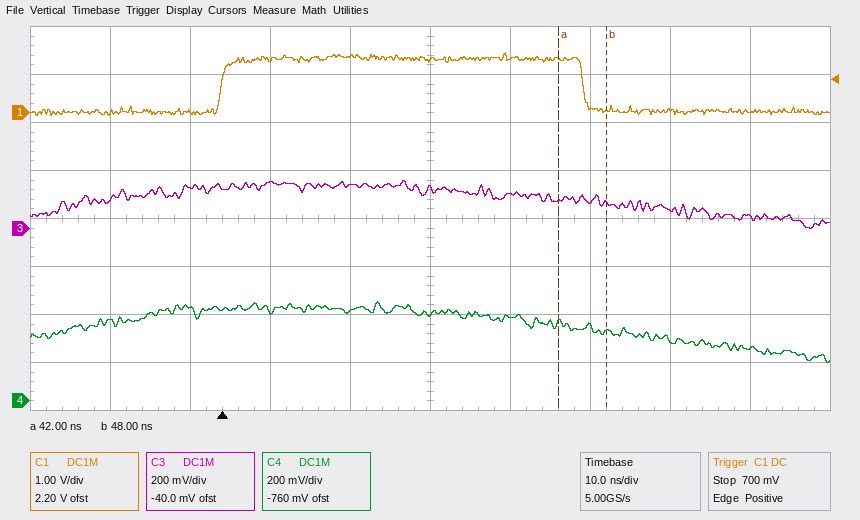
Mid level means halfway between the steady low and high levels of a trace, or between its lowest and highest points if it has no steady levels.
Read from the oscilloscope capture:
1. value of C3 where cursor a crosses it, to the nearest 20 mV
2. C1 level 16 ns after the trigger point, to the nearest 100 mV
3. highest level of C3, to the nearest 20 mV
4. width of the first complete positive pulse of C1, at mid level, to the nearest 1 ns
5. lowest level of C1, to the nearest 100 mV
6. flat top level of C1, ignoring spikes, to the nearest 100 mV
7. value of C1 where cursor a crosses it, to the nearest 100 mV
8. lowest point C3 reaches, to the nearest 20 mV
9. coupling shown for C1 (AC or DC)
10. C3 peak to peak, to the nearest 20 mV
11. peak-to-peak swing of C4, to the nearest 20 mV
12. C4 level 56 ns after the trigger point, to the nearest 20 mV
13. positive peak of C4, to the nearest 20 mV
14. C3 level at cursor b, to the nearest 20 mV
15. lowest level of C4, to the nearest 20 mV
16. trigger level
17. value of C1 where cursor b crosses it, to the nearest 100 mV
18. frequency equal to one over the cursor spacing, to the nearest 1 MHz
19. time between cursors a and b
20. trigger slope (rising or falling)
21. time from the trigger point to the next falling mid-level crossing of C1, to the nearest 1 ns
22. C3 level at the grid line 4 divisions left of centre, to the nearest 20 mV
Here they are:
120 mV
1.2 V
200 mV
45 ns
-100 mV
1.1 V
1.1 V
0 mV
DC
200 mV
260 mV
260 mV
420 mV
100 mV
160 mV
700 mV
0.0 V
167 MHz
6 ns
rising
45 ns
120 mV
